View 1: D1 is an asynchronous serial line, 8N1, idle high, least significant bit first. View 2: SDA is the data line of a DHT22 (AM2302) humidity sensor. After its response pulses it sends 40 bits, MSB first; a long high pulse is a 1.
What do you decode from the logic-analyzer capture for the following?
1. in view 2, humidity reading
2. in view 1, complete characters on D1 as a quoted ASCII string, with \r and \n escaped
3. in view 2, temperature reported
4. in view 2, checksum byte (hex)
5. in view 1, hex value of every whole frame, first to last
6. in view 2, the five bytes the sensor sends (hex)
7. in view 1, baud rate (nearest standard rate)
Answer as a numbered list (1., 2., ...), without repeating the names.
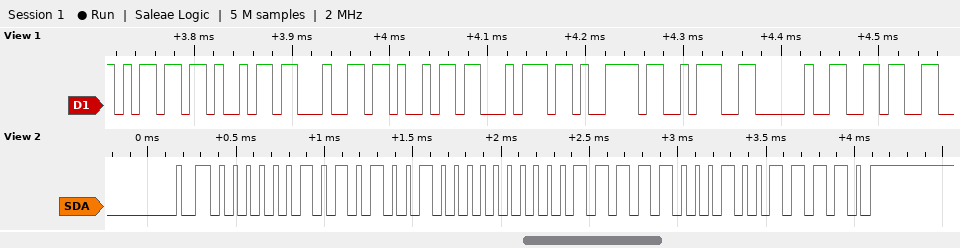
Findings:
1. 67.6 %
2. "midity: 6"
3. 24.8 °C
4. 0x9E
5. 0x6D 0x69 0x64 0x69 0x74 0x79 0x3A 0x20 0x36
6. 02 A4 00 F8 9E
7. 115200 baud
